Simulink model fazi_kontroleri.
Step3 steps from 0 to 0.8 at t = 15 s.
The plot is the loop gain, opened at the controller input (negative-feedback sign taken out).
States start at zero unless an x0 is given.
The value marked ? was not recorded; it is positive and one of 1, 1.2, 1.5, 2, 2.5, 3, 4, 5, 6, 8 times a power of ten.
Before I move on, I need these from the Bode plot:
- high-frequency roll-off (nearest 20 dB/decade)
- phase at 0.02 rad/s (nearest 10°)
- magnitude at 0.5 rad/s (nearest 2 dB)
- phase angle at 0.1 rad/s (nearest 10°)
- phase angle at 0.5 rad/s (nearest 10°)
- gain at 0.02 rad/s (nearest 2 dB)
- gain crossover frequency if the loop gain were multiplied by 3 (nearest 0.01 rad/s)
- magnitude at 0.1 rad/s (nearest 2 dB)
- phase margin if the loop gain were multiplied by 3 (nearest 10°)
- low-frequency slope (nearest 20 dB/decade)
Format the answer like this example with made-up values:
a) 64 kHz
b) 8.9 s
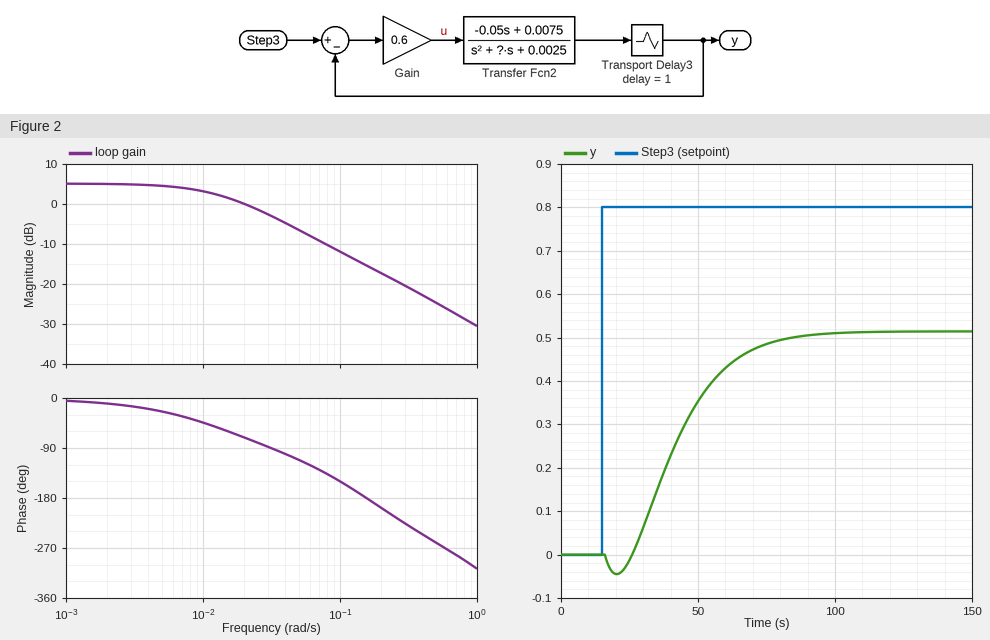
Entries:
a) -20 dB/decade
b) -70°
c) -24 dB
d) -150°
e) -260°
f) 0 dB
g) 0.07 rad/s
h) -12 dB
i) 50°
j) 0 dB/decade
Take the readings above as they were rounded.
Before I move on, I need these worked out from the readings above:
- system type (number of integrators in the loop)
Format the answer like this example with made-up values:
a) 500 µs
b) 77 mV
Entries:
a) 0
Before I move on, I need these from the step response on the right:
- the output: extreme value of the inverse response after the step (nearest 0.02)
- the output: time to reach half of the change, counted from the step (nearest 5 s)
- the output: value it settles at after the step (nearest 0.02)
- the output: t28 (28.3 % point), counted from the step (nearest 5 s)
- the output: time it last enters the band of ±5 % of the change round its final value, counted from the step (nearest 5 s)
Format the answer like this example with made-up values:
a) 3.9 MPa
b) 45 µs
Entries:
a) -0.04
b) 25 s
c) 0.52
d) 20 s
e) 60 s
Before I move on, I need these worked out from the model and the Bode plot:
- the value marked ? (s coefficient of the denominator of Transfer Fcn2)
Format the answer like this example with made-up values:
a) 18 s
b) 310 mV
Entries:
a) 0.2
